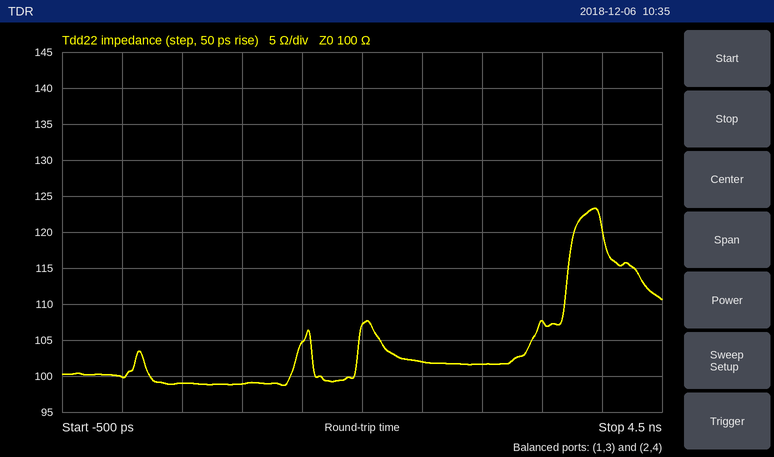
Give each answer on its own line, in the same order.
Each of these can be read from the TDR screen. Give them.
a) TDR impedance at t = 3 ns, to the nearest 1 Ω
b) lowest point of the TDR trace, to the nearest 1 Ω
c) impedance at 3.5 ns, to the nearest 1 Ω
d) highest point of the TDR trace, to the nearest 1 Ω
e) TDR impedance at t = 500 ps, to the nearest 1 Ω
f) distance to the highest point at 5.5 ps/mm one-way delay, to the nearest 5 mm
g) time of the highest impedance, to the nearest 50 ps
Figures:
102 Ω
99 Ω
108 Ω
123 Ω
99 Ω
360 mm
3.95 ns
